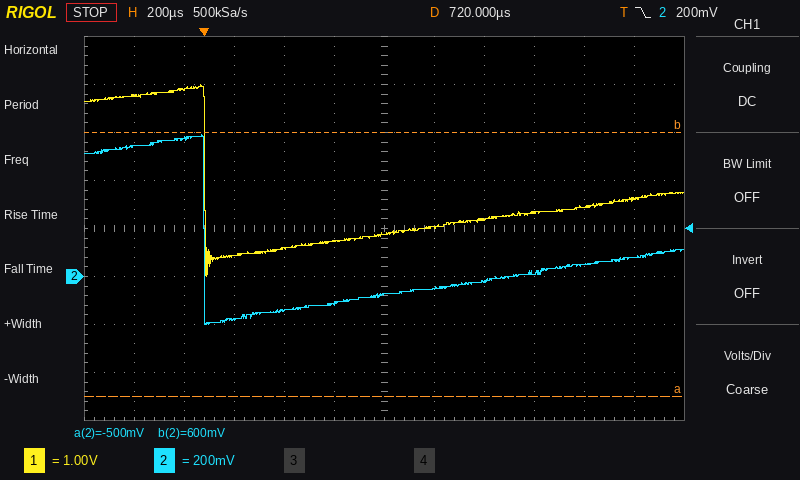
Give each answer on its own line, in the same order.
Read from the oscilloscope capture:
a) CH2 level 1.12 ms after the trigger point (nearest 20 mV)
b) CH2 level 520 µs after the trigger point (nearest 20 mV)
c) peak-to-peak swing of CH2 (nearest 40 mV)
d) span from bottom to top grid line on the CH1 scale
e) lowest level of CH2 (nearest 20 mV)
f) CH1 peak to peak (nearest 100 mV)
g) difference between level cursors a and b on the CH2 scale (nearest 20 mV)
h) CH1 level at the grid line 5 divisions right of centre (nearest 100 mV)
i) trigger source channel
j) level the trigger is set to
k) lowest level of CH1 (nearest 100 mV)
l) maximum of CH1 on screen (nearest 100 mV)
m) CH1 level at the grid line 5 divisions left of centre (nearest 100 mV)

-20 mV
-120 mV
800 mV
8 V
-200 mV
4.0 V
1.10 V
1.6 V
CH2
200 mV
0.0 V
4.0 V
3.8 V
